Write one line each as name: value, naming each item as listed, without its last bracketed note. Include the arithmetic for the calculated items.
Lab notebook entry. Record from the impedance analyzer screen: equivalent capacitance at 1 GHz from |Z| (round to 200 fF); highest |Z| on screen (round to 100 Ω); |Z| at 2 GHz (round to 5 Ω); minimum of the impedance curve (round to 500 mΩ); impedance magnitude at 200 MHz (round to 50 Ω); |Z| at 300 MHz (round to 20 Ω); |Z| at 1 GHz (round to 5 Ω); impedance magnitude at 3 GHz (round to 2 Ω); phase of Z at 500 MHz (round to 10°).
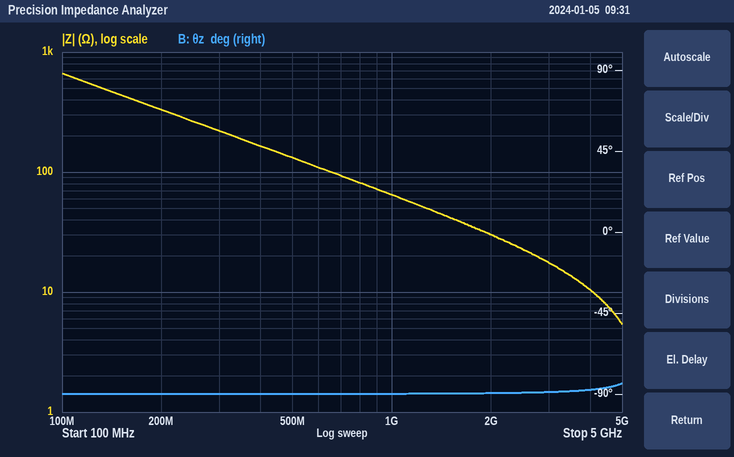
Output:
equivalent capacitance at 1 GHz from |Z|: C = 1/(2π × 1 GHz × 65 Ω) ≈ 2.4 pF
highest |Z| on screen: 700 Ω
|Z| at 2 GHz: 30 Ω
minimum of the impedance curve: 5.5 Ω
impedance magnitude at 200 MHz: 350 Ω
|Z| at 300 MHz: 220 Ω
|Z| at 1 GHz: 65 Ω
impedance magnitude at 3 GHz: 18 Ω
phase of Z at 500 MHz: -90°
